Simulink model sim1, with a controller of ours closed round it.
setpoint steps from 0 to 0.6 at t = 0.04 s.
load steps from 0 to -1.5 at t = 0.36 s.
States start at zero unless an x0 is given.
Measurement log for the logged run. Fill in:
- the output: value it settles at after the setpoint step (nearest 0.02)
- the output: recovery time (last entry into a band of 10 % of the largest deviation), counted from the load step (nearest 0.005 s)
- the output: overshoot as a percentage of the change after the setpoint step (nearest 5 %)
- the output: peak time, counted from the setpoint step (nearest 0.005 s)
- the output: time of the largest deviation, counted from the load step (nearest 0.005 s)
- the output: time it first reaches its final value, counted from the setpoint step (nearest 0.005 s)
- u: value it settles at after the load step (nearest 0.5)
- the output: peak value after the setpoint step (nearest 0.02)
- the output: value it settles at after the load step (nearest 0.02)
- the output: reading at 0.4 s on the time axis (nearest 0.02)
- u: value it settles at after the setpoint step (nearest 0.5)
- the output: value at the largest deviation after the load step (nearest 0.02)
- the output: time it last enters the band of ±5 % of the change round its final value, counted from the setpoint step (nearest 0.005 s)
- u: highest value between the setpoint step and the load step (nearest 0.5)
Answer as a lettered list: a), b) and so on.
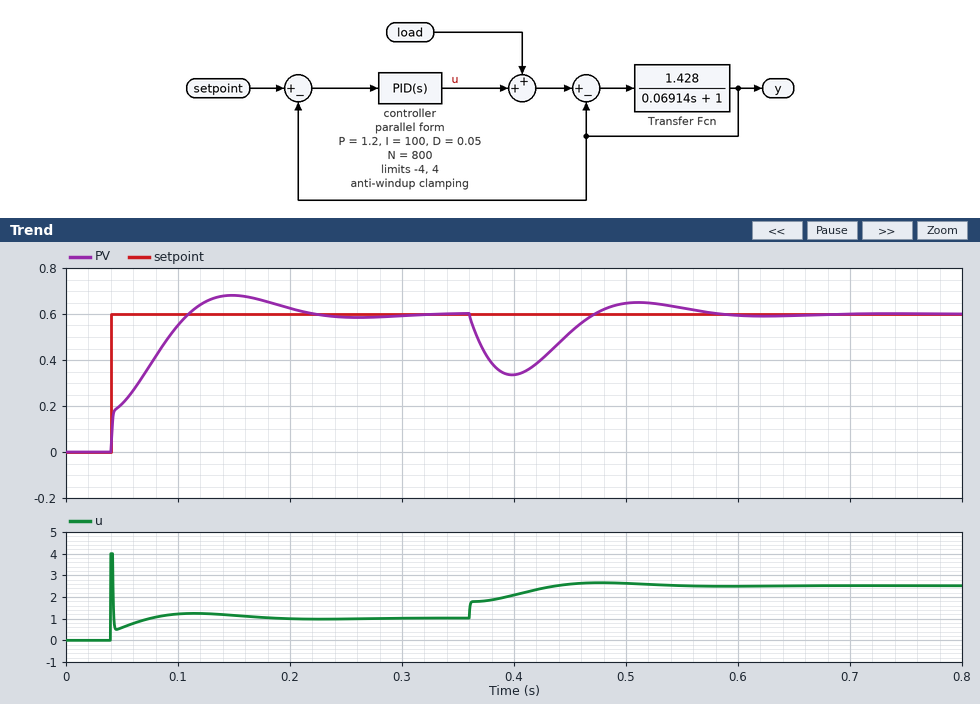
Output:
a) 0.60
b) 0.190 s
c) 15 %
d) 0.110 s
e) 0.040 s
f) 0.070 s
g) 2.5
h) 0.68
i) 0.60
j) 0.34
k) 1.0
l) 0.34
m) 0.155 s
n) 4.0
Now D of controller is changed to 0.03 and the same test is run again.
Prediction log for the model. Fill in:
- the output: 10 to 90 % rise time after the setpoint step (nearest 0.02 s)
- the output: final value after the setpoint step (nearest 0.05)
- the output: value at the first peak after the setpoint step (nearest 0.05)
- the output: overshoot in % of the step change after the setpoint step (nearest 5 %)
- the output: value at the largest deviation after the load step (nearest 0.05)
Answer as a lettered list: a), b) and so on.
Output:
a) 0.06 s
b) 0.60
c) 0.65
d) 10 %
e) 0.30
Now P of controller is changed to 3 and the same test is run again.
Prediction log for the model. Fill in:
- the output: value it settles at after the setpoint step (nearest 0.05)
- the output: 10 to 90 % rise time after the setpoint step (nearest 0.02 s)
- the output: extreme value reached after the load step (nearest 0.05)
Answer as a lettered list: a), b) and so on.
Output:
a) 0.60
b) 0.06 s
c) 0.40
